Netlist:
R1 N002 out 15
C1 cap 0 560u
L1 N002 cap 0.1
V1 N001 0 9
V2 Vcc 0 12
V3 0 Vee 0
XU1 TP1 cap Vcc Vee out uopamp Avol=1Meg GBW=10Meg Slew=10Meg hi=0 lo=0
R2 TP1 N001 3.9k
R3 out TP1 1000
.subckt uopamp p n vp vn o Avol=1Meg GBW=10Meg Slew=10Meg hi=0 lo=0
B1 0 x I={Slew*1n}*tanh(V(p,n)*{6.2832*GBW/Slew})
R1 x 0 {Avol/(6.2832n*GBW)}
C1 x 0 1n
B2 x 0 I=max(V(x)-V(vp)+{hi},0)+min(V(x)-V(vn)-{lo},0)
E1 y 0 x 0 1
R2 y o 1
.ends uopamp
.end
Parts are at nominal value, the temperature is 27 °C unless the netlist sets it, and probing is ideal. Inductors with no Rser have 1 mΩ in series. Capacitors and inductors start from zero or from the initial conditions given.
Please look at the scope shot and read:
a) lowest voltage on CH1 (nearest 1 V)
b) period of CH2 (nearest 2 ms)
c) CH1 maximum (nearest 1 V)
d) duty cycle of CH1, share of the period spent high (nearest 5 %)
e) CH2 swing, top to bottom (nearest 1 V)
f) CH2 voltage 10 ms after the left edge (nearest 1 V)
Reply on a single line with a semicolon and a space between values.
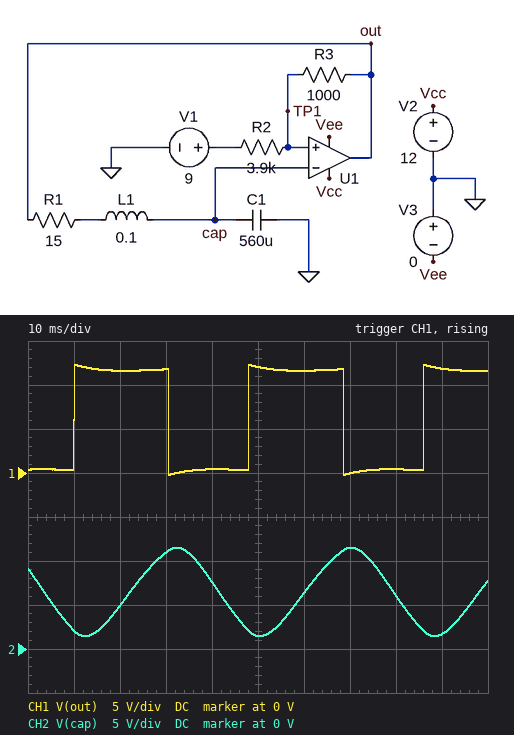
0 V; 38 ms; 12 V; 55 %; 10 V; 2 V
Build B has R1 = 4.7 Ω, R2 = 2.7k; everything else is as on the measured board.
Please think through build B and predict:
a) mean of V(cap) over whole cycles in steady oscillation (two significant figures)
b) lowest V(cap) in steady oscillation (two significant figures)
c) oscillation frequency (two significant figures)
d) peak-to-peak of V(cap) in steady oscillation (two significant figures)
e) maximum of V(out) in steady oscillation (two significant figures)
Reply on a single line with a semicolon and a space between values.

6.4 V; -640 mV; 29 Hz; 14 V; 13 V
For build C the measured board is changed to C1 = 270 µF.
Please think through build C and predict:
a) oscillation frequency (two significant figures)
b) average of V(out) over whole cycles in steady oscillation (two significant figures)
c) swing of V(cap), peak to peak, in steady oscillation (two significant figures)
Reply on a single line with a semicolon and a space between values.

41 Hz; 6.4 V; 11 V
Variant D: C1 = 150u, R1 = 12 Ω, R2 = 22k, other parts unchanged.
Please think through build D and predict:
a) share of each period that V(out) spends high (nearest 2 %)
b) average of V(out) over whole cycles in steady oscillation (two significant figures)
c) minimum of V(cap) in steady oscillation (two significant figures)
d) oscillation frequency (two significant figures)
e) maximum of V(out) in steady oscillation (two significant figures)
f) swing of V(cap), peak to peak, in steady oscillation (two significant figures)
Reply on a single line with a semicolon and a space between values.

50 %; 6.1 V; -1.9 V; 54 Hz; 12 V; 16 V
